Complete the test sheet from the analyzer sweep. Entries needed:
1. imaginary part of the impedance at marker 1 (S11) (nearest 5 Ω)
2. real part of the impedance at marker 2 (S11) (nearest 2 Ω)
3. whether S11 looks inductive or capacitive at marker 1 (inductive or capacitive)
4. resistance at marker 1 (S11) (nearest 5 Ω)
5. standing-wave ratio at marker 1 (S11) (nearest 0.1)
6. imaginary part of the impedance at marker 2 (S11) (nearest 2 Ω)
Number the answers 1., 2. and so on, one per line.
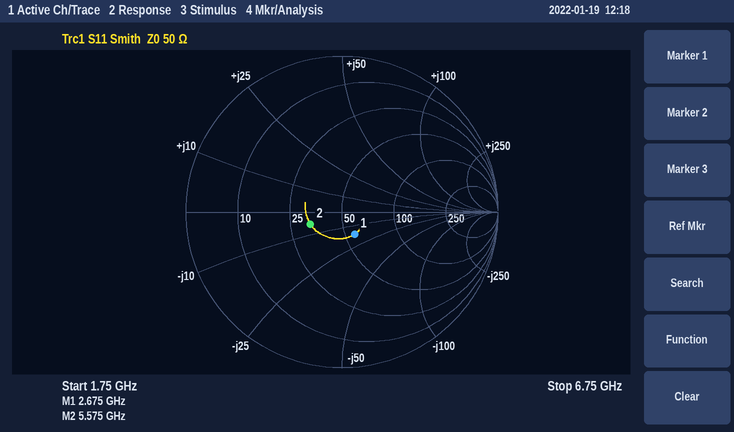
1. -15 Ω
2. 32 Ω
3. capacitive
4. 55 Ω
5. 1.4
6. -6 Ω
